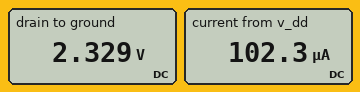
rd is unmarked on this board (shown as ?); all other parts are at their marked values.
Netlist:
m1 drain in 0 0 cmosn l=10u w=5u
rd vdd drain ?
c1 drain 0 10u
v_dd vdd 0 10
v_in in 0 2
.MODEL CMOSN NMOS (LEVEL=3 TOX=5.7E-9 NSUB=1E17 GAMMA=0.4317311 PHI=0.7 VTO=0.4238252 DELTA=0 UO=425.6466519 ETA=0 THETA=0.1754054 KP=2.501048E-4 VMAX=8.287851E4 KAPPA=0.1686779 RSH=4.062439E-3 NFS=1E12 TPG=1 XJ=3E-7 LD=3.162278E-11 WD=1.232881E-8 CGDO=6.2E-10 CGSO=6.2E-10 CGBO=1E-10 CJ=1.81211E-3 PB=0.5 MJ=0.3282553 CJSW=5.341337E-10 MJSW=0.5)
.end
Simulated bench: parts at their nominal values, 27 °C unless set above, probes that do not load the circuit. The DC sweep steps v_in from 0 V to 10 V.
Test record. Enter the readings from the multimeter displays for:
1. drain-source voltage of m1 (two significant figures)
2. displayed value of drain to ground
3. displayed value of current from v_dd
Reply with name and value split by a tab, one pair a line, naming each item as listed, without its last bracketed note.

drain-source voltage of m1	2.3 V
displayed value of drain to ground	2.329 V
displayed value of current from v_dd	102.3 µA
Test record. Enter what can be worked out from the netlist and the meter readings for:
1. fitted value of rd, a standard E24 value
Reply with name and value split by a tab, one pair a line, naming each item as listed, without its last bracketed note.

fitted value of rd, a standard E24 value	75 kΩ
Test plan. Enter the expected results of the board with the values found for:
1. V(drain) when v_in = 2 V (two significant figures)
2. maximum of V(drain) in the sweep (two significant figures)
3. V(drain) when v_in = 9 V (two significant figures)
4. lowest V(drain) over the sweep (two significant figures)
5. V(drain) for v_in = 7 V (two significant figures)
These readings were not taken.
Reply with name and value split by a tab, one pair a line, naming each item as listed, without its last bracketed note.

V(drain) when v_in = 2 V	2.3 V
maximum of V(drain) in the sweep	10 V
V(drain) when v_in = 9 V	310 mV
lowest V(drain) over the sweep	300 mV
V(drain) for v_in = 7 V	350 mV
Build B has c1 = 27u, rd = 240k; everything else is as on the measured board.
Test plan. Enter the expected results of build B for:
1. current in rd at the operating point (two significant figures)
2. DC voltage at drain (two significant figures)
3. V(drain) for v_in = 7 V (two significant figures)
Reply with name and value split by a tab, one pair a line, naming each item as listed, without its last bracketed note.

current in rd at the operating point	40 µA
DC voltage at drain	300 mV
V(drain) for v_in = 7 V	110 mV
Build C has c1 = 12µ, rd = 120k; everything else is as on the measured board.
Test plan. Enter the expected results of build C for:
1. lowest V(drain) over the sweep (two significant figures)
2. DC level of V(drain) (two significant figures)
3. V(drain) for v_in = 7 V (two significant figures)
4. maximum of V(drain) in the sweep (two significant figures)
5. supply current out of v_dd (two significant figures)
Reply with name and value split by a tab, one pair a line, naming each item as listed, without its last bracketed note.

lowest V(drain) over the sweep	190 mV
DC level of V(drain)	690 mV
V(drain) for v_in = 7 V	220 mV
maximum of V(drain) in the sweep	10 V
supply current out of v_dd	78 µA
